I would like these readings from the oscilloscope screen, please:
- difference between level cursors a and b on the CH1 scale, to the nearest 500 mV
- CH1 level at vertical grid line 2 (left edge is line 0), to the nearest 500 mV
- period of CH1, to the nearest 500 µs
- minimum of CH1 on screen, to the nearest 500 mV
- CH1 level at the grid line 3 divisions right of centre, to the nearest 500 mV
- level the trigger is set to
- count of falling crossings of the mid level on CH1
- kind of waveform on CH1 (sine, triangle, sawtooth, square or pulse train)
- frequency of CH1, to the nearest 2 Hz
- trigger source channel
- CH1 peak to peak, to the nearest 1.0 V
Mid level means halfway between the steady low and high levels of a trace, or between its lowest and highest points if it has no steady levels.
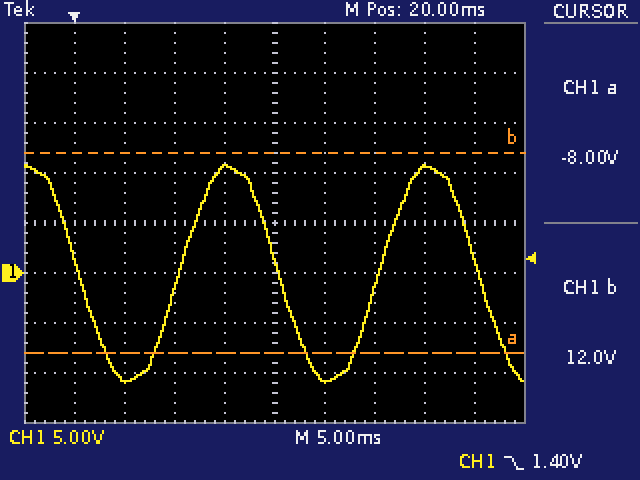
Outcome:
20.0 V
-10.5 V
20.0 ms
-11.0 V
10.5 V
1.40 V
3
sine
50 Hz
CH1
22.0 V
